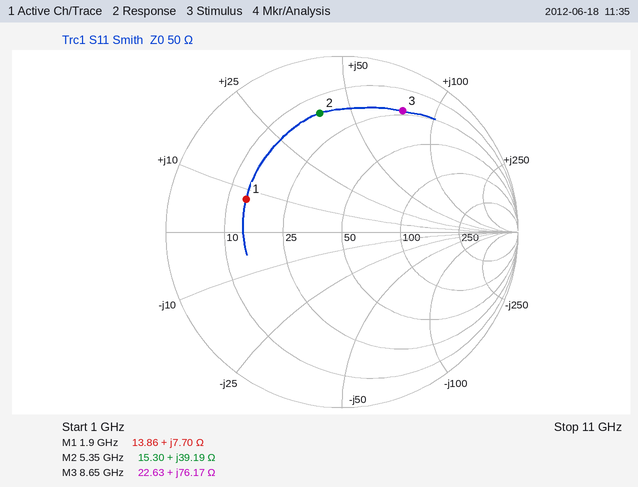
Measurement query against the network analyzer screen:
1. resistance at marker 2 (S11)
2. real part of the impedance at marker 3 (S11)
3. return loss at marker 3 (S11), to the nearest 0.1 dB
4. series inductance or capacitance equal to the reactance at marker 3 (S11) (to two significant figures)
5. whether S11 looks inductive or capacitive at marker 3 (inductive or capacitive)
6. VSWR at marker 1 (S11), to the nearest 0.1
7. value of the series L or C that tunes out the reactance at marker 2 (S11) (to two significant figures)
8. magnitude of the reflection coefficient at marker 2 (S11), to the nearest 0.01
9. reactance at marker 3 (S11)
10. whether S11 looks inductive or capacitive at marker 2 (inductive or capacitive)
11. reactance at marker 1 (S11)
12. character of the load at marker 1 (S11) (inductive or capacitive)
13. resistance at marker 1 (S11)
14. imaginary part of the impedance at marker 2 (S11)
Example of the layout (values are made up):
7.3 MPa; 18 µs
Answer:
15.30 Ω; 22.63 Ω; 2.3 dB; 1.4 nH; inductive; 3.7; 760 fF; 0.69; +76.17 Ω; inductive; +7.70 Ω; inductive; 13.86 Ω; +39.19 Ω
